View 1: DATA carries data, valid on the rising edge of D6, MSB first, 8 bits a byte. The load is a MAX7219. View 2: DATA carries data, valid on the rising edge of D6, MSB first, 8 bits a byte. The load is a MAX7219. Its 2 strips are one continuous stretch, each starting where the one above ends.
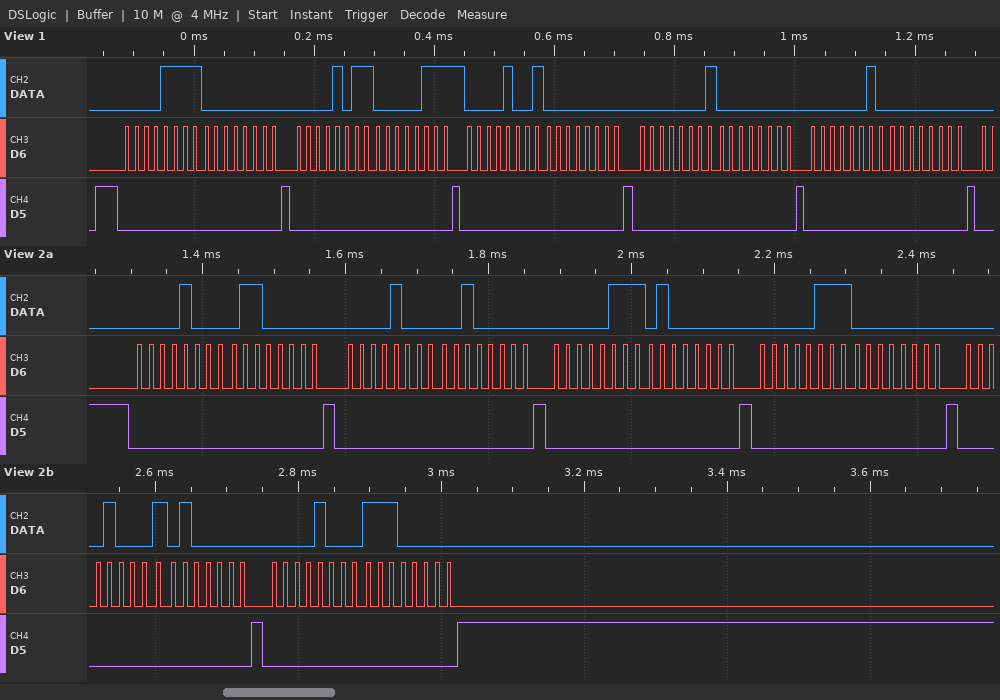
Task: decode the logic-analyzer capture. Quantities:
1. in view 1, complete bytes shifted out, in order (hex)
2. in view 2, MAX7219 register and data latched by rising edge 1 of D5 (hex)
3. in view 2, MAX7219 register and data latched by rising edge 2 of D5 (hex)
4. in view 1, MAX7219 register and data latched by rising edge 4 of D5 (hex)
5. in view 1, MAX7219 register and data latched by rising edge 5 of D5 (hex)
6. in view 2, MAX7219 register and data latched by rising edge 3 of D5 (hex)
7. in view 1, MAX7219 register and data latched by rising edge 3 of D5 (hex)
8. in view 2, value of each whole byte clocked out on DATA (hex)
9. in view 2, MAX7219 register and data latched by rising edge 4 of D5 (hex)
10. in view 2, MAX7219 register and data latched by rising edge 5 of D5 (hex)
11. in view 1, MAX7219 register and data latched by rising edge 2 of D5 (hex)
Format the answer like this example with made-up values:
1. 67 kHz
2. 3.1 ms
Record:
1. 0x0F 0x00 0x0B 0x07 0x09 0x00 0x01 0x00 0x02 0x00
2. register 0x8, data 0x60
3. register 0x8, data 0x20
4. register 0x9, data 0x00
5. register 0x1, data 0x00
6. register 0x7, data 0x40
7. register 0xB, data 0x07
8. 08 60 08 20 07 40 07 00 08 A0 08 E0
9. register 0x7, data 0x00
10. register 0x8, data 0xA0
11. register 0xF, data 0x00
